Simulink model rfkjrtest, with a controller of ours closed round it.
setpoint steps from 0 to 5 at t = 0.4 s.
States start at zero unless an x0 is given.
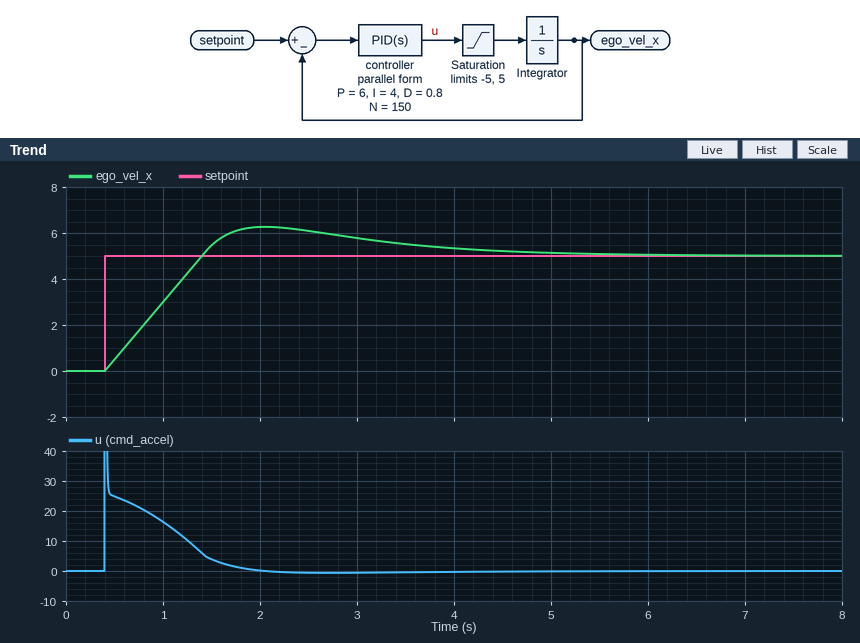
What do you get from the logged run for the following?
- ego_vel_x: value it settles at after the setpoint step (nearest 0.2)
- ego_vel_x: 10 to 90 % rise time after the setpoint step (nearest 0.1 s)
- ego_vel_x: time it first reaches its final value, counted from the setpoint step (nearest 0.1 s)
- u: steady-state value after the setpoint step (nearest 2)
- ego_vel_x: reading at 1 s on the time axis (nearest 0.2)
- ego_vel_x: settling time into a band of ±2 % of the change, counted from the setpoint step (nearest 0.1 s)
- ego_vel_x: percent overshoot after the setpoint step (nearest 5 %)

5.0
0.8 s
1.0 s
0
3.0
4.9 s
25 %
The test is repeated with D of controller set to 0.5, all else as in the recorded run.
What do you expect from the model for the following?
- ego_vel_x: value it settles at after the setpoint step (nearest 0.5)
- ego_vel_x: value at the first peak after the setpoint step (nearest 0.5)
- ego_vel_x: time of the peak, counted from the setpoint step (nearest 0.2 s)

5.0
6.5
1.6 s
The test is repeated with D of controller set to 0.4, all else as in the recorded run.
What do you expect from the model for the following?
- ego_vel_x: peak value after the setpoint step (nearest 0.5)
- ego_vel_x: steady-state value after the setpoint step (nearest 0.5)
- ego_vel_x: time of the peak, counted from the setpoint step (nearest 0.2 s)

6.5
5.0
1.6 s
